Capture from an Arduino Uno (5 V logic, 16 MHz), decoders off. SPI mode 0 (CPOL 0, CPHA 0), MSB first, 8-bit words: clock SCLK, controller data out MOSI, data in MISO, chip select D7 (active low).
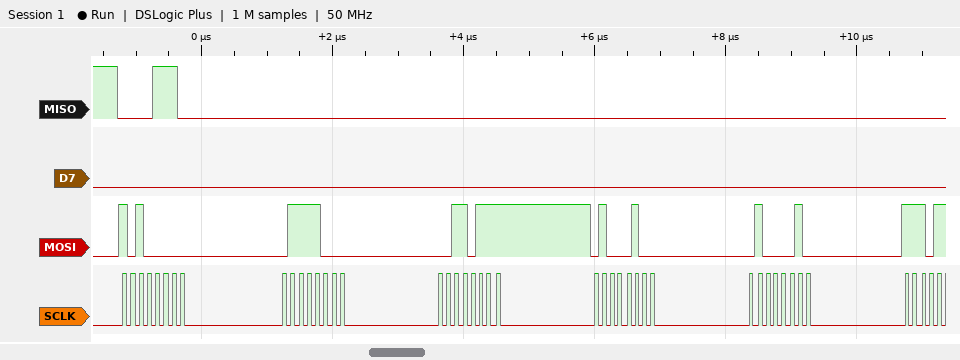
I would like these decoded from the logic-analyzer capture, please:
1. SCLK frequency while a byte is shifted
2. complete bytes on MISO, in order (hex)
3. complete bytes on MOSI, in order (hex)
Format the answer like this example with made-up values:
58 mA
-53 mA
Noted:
8 MHz
0E 00 00 00 00
A0 78 37 44 42
